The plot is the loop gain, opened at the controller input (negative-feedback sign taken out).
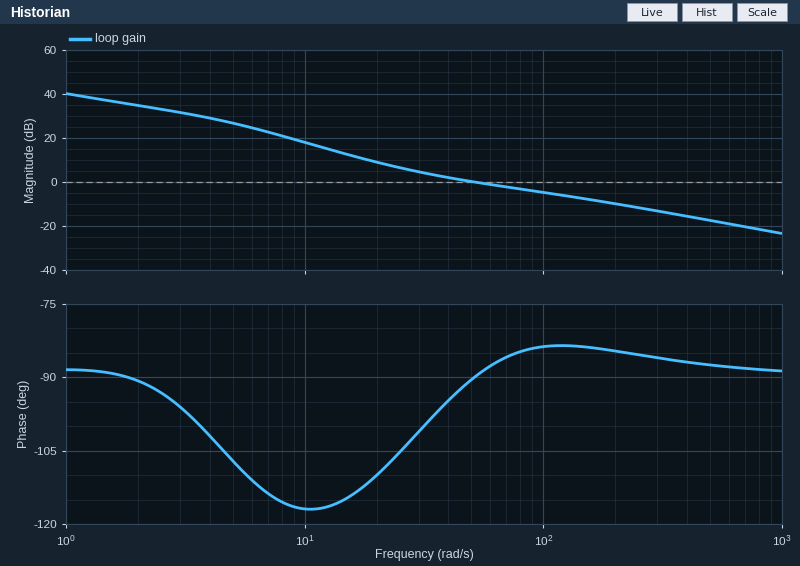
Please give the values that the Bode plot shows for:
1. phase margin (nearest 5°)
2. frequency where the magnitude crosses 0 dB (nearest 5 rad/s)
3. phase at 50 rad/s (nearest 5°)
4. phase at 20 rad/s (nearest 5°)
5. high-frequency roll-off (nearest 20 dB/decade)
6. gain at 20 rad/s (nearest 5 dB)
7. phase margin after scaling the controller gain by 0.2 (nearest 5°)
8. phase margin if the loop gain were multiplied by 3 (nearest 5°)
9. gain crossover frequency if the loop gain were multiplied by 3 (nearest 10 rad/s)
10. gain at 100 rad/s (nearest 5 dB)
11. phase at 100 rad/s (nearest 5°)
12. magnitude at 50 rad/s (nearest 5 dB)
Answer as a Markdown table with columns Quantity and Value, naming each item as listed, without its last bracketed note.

| Quantity | Value |
|---|---|
| phase margin | 90° |
| frequency where the magnitude crosses 0 dB | 50 rad/s |
| phase at 50 rad/s | -90° |
| phase at 20 rad/s | -110° |
| high-frequency roll-off | -20 dB/decade |
| gain at 20 rad/s | 10 dB |
| phase margin after scaling the controller gain by 0.2 | 65° |
| phase margin if the loop gain were multiplied by 3 | 95° |
| gain crossover frequency if the loop gain were multiplied by 3 | 190 rad/s |
| gain at 100 rad/s | -5 dB |
| phase at 100 rad/s | -85° |
| magnitude at 50 rad/s | 0 dB |
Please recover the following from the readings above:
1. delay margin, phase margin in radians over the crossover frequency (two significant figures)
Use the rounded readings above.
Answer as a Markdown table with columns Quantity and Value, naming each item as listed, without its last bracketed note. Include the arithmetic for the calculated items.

| Quantity | Value |
|---|---|
| delay margin, phase margin in radians over the crossover frequency | 90 × π / 180 / 50 = 0.031 s |
